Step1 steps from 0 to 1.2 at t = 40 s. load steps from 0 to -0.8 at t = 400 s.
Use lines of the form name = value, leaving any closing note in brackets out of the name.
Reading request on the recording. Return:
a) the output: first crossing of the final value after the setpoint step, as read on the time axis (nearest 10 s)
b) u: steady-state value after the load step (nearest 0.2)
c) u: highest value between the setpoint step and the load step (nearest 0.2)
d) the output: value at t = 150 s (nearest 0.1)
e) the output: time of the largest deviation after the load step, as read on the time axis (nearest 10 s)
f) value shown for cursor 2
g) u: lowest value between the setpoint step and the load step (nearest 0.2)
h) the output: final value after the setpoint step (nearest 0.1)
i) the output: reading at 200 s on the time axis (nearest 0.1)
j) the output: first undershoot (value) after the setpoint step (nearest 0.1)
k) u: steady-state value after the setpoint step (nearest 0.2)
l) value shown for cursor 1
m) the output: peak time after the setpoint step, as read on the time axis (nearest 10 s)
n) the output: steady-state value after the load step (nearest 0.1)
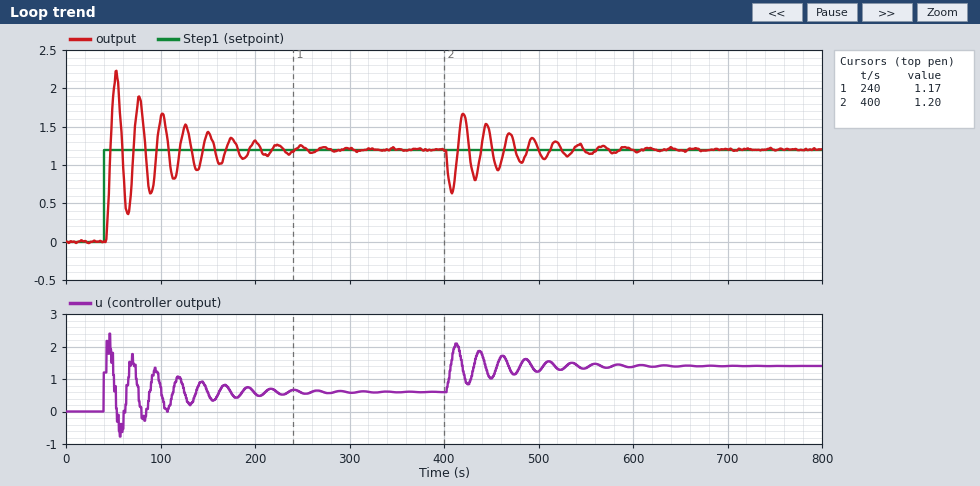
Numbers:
the output: first crossing of the final value after the setpoint step, as read on the time axis = 50 s
u: steady-state value after the load step = 1.4
u: highest value between the setpoint step and the load step = 2.4
the output: value at t = 150 s = 1.4
the output: time of the largest deviation after the load step, as read on the time axis = 410 s
value shown for cursor 2 = 1.20
u: lowest value between the setpoint step and the load step = -0.8
the output: final value after the setpoint step = 1.2
the output: reading at 200 s on the time axis = 1.3
the output: first undershoot (value) after the setpoint step = 0.4
u: steady-state value after the setpoint step = 0.6
value shown for cursor 1 = 1.17
the output: peak time after the setpoint step, as read on the time axis = 50 s
the output: steady-state value after the load step = 1.2
